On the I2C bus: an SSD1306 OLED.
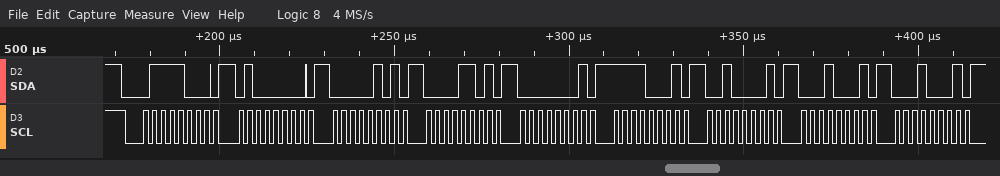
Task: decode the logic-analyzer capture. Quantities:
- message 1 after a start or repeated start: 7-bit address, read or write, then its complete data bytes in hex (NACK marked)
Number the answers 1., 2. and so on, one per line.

1. 0x3C write: 40 05 0D 01 F1 21 11 11
